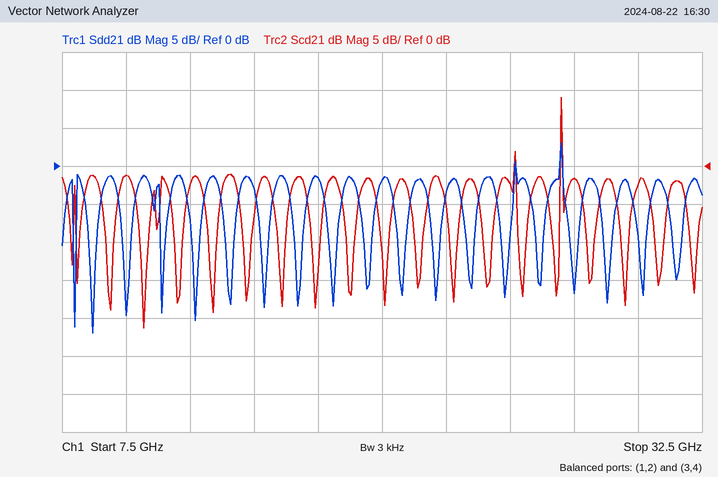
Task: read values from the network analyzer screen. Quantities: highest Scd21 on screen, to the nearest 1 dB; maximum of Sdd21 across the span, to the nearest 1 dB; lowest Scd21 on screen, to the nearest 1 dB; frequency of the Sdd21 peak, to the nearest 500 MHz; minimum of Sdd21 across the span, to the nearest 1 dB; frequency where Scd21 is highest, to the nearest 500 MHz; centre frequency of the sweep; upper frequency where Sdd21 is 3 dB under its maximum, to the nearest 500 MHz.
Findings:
9 dB
3 dB
-21 dB
27.0 GHz
-22 dB
27.0 GHz
20 GHz
27.0 GHz
